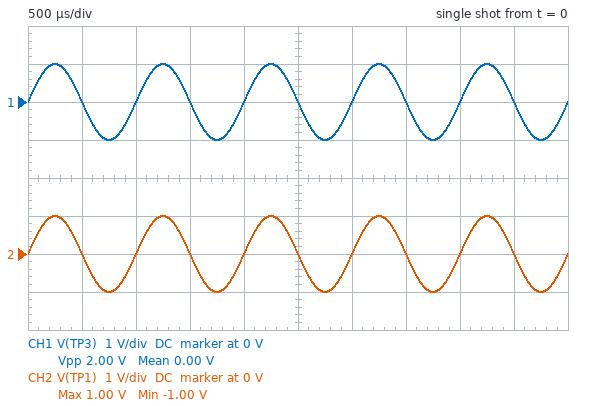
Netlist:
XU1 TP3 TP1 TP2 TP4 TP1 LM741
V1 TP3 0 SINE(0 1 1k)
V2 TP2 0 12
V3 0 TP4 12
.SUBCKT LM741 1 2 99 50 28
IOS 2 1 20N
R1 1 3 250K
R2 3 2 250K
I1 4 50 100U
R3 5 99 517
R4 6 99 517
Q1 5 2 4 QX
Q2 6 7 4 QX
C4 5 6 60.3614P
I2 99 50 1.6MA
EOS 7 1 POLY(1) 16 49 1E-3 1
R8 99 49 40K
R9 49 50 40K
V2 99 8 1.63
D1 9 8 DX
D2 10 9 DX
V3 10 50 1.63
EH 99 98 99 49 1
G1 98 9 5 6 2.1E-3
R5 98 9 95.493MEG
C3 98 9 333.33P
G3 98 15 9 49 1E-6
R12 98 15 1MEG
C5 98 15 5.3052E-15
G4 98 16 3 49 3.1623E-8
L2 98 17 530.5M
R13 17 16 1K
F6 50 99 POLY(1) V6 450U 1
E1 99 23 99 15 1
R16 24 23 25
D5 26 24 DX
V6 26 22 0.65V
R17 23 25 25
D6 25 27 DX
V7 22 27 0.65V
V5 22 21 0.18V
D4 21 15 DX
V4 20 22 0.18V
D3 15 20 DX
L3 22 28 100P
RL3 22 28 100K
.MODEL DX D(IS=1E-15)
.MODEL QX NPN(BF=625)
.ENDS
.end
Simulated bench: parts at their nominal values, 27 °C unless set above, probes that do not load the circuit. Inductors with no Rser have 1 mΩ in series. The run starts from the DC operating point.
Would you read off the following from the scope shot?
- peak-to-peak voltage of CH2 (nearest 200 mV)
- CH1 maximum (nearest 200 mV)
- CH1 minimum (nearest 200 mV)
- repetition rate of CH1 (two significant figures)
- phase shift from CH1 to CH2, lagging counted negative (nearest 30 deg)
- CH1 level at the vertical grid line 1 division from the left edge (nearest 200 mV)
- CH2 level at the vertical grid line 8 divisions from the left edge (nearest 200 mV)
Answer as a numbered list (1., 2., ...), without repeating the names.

1. 2.0 V
2. 1.0 V
3. -1.0 V
4. 1.0 kHz
5. 0 deg
6. 0 V
7. 0 V
